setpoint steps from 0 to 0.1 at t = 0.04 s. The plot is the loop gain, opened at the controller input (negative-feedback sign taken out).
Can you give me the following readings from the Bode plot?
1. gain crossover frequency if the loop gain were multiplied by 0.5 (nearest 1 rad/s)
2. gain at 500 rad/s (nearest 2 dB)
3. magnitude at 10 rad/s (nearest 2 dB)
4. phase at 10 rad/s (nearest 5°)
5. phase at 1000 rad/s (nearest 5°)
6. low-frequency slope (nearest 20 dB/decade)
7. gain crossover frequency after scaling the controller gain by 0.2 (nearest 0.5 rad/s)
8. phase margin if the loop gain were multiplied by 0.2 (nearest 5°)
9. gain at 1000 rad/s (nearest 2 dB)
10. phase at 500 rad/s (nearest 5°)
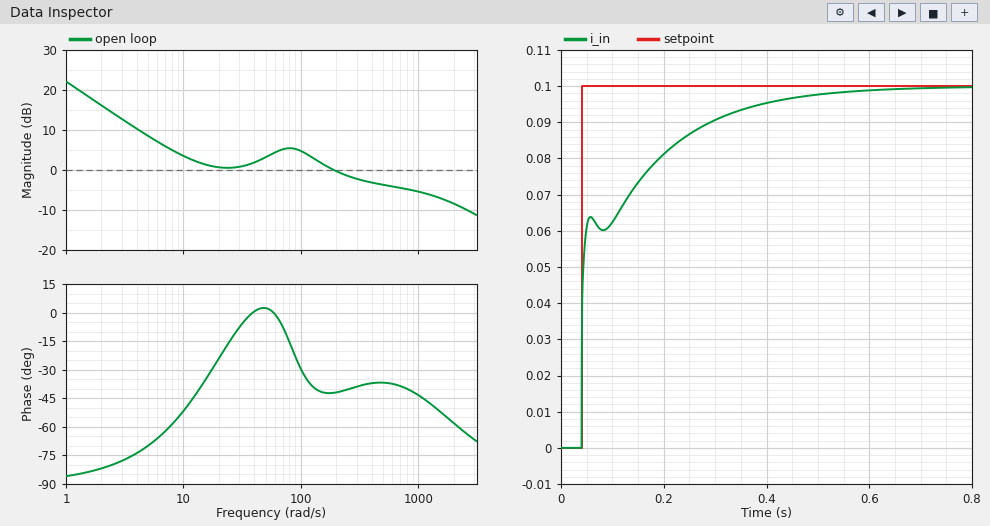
7 rad/s
-4 dB
4 dB
-50°
-45°
-20 dB/decade
2.5 rad/s
100°
-6 dB
-35°
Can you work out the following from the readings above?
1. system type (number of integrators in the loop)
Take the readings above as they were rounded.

1
